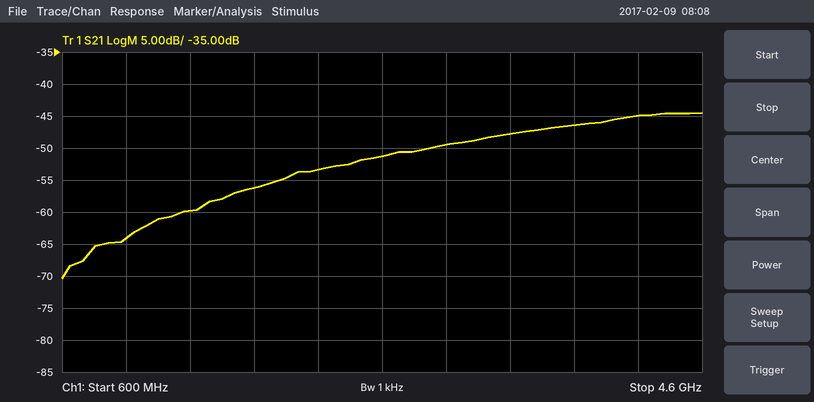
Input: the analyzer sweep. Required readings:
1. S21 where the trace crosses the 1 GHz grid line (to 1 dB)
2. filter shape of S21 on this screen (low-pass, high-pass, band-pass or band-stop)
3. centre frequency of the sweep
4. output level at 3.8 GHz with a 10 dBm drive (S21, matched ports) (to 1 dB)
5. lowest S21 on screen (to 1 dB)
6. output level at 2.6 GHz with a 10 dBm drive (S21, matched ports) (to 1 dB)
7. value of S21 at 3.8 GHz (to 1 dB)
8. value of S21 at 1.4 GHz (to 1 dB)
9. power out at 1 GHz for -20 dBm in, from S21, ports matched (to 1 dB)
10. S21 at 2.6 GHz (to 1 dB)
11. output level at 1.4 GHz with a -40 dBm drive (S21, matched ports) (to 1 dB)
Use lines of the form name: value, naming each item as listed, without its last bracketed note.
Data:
S21 where the trace crosses the 1 GHz grid line: -64 dB
filter shape of S21 on this screen: high-pass
centre frequency of the sweep: 2.6 GHz
output level at 3.8 GHz with a 10 dBm drive (S21, matched ports): -36 dBm
lowest S21 on screen: -70 dB
output level at 2.6 GHz with a 10 dBm drive (S21, matched ports): -41 dBm
value of S21 at 3.8 GHz: -46 dB
value of S21 at 1.4 GHz: -60 dB
power out at 1 GHz for -20 dBm in, from S21, ports matched: -84 dBm
S21 at 2.6 GHz: -51 dB
output level at 1.4 GHz with a -40 dBm drive (S21, matched ports): -100 dBm
